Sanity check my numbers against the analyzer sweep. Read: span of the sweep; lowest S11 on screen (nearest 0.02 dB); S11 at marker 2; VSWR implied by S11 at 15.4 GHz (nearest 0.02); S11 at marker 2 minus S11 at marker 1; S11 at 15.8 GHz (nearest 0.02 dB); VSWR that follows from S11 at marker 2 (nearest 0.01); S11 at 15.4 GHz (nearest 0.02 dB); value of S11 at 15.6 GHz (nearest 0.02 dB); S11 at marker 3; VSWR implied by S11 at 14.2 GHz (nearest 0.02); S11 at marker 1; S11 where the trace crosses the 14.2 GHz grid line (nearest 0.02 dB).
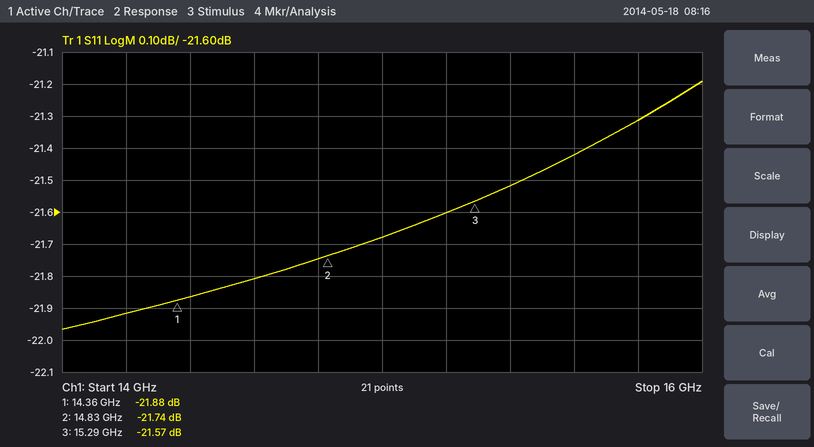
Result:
2 GHz
-21.96 dB
-21.74 dB
1.18
0.14 dB
-21.32 dB
1.18
-21.52 dB
-21.42 dB
-21.57 dB
1.18
-21.88 dB
-21.92 dB
